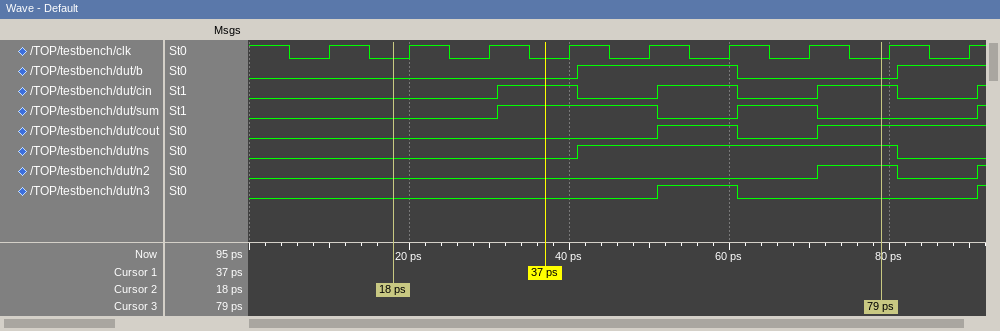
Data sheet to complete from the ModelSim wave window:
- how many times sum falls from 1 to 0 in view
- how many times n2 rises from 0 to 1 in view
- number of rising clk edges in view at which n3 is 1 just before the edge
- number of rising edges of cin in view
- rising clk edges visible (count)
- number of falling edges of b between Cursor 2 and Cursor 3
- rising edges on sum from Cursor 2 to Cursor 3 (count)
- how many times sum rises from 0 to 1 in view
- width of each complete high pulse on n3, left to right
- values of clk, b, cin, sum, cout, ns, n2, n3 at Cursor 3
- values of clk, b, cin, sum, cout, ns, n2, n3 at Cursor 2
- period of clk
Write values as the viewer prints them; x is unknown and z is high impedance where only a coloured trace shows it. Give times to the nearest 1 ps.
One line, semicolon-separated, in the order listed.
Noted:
2; 2; 1; 4; 9; 1; 2; 3; 10 ps; clk=0, b=0, cin=1, sum=0, cout=1, ns=1, n2=1, n3=0; clk=0, b=0, cin=0, sum=0, cout=0, ns=0, n2=0, n3=0; 10 ps
